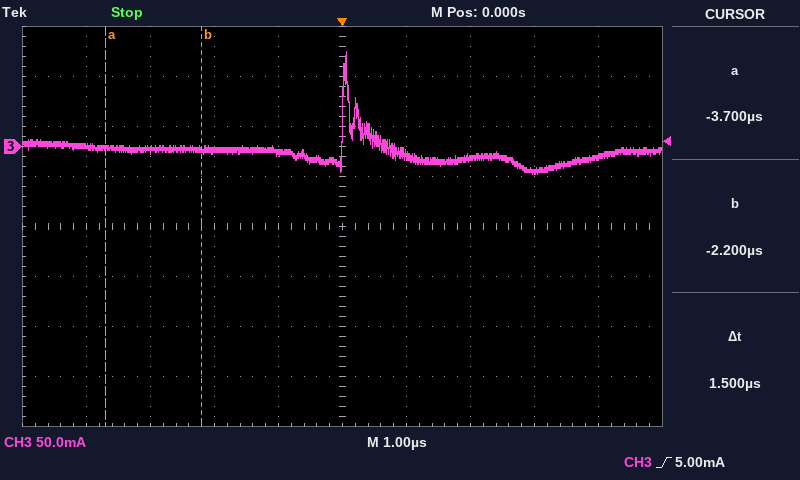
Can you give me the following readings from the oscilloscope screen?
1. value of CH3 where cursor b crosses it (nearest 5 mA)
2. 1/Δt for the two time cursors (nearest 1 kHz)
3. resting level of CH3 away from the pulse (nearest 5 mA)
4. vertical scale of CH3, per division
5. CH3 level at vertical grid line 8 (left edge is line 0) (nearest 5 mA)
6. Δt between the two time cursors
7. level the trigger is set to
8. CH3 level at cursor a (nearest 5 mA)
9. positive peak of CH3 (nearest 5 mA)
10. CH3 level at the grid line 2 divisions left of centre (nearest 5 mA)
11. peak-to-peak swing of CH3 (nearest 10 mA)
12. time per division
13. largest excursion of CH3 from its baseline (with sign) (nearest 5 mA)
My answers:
-5 mA
667 kHz
-5 mA
50 mA
-25 mA
1.5 µs
5.00 mA
0 mA
95 mA
-5 mA
120 mA
1 µs
+100 mA
